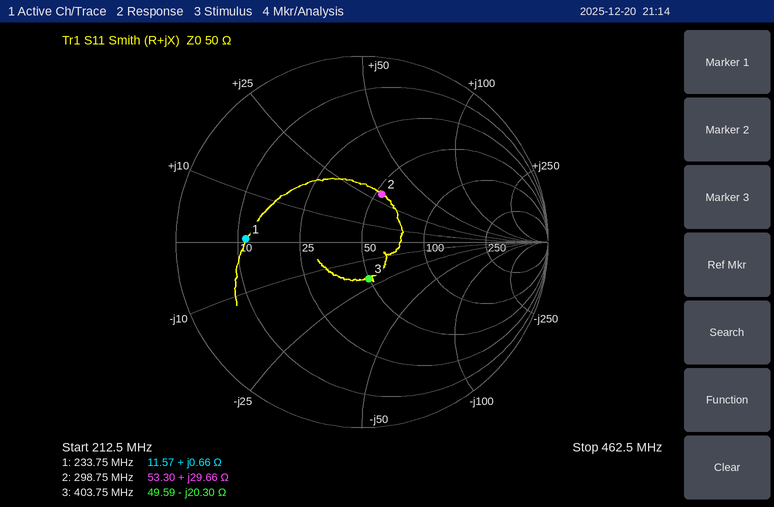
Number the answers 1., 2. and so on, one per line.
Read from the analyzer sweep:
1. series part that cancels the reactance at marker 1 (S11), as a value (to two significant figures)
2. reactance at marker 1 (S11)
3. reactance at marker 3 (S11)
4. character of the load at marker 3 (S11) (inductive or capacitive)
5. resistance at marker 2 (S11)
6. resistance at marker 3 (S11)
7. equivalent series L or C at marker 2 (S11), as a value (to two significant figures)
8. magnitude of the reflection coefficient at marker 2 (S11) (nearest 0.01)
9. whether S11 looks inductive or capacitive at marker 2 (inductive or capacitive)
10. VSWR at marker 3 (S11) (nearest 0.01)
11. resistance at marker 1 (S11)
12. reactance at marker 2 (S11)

1. 1.0 nF
2. +0.66 Ω
3. -20.30 Ω
4. capacitive
5. 53.30 Ω
6. 49.59 Ω
7. 16 nH
8. 0.28
9. inductive
10. 1.50
11. 11.57 Ω
12. +29.66 Ω
